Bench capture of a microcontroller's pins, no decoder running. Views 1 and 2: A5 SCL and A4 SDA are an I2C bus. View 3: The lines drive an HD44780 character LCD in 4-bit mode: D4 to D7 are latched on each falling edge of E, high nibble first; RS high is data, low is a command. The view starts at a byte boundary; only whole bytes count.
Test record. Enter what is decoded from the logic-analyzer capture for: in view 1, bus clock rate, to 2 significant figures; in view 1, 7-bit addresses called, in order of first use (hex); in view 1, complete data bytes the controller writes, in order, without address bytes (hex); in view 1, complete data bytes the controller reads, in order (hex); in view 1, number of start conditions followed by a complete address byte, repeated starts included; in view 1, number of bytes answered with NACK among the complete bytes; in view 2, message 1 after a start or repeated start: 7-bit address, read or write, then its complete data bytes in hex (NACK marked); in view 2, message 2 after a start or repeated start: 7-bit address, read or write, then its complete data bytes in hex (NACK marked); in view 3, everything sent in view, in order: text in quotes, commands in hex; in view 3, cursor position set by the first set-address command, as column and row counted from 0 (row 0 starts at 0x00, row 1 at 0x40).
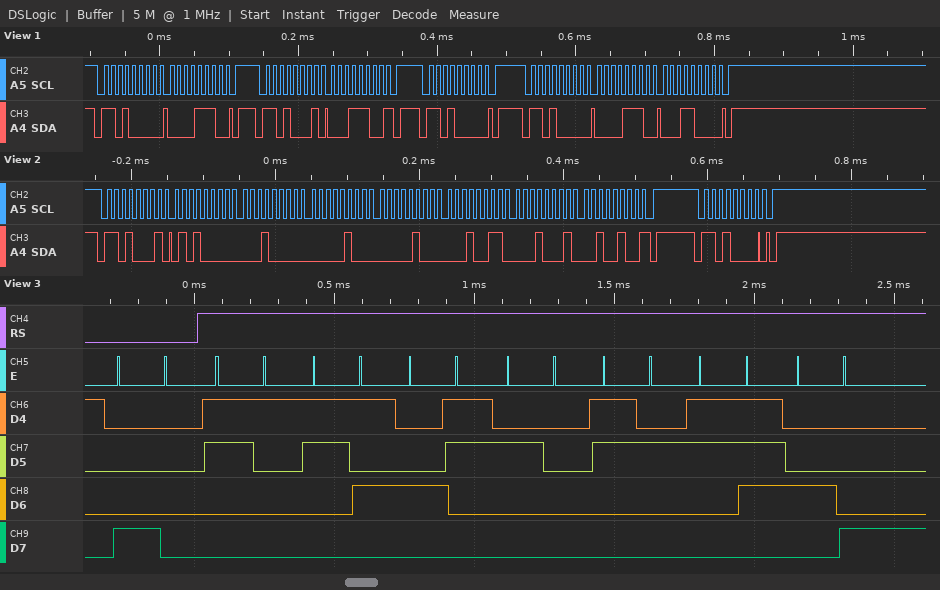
100 kHz
0x68
0E 0E 18
1C
4
1
0x68 read: 50 10 04 04 13 11 24 NACK
0x68 write
0x80 "15C 27H"
column 0, row 0
